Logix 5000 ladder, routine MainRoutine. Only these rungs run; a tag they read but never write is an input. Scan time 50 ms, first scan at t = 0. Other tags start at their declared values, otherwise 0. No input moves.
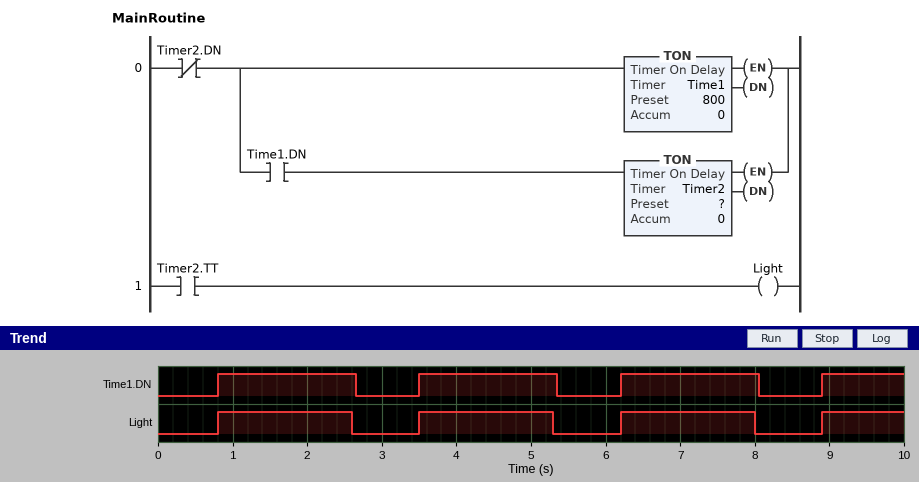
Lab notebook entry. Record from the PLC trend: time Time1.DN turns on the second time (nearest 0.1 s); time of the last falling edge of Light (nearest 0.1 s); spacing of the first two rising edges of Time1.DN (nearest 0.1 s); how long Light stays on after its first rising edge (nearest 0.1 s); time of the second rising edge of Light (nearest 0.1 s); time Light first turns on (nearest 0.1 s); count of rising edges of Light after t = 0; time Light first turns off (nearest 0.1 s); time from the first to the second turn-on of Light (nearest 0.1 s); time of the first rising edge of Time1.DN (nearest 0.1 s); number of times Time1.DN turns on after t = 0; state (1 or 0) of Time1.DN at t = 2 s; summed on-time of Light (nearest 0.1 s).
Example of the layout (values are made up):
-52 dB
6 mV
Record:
3.5 s
8.0 s
2.7 s
1.8 s
3.5 s
0.8 s
4
2.6 s
2.7 s
0.8 s
4
1
6.5 s
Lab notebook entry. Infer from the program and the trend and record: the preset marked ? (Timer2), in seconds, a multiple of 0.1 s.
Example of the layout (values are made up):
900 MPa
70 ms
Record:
1.8 s
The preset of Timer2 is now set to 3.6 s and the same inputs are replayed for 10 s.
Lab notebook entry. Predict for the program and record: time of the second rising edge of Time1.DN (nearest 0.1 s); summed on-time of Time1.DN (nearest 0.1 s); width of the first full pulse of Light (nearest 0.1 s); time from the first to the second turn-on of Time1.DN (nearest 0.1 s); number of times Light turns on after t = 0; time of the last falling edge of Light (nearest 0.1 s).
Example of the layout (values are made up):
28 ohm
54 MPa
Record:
5.3 s
7.5 s
3.6 s
4.5 s
3
8.9 s
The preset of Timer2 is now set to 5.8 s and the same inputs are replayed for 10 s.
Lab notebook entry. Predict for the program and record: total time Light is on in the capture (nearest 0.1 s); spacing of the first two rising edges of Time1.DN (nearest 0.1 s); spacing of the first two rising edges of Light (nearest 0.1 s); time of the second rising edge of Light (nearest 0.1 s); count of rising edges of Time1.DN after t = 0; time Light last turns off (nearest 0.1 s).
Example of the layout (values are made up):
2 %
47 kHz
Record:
8.3 s
6.7 s
6.7 s
7.5 s
2
6.6 s
